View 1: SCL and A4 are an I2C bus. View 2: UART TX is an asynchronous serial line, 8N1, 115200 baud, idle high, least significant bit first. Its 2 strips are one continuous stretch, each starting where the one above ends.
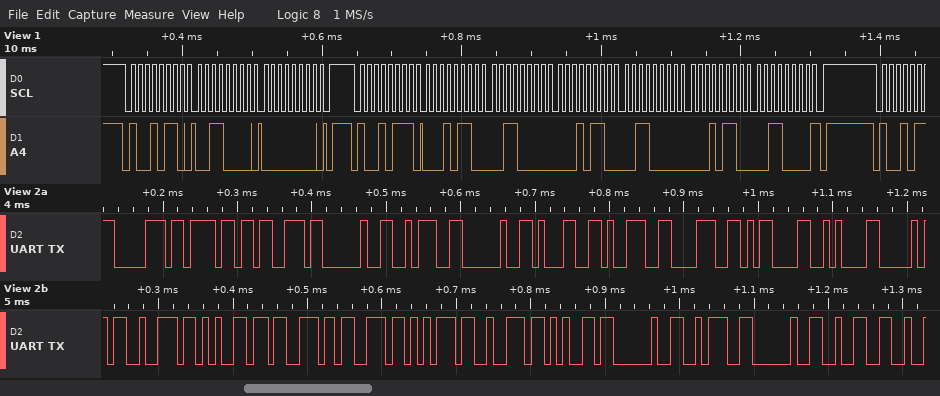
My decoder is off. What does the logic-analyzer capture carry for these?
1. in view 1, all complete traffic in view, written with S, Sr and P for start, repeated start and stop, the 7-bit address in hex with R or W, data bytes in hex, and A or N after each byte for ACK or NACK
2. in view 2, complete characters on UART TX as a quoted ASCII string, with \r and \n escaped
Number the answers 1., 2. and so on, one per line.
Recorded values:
1. S 4BW A 30 A 00 A P S 4BR A 16 A 30 A 16 A 30 A 16 A 30 N P
2. "pos : 198\r\nPressure : 2"
